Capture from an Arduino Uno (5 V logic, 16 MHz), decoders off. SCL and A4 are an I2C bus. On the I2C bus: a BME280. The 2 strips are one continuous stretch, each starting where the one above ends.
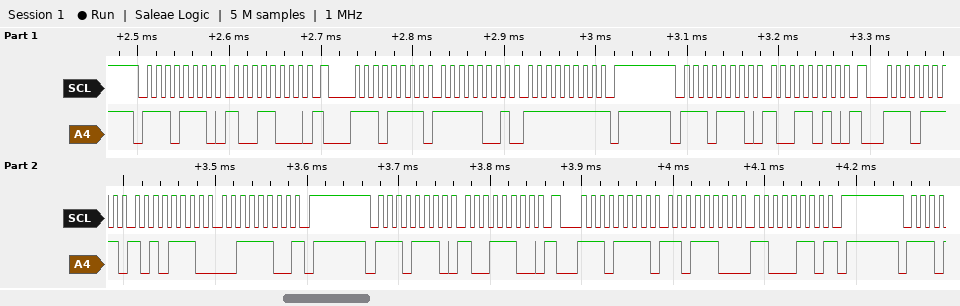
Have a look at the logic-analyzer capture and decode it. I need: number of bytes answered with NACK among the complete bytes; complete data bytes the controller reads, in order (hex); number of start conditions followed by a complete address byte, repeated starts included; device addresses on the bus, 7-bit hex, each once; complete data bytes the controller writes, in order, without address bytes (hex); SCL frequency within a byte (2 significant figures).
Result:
3
F9 FF AE 3C DC C6
6
0x77
98 9A 9C
100 kHz
